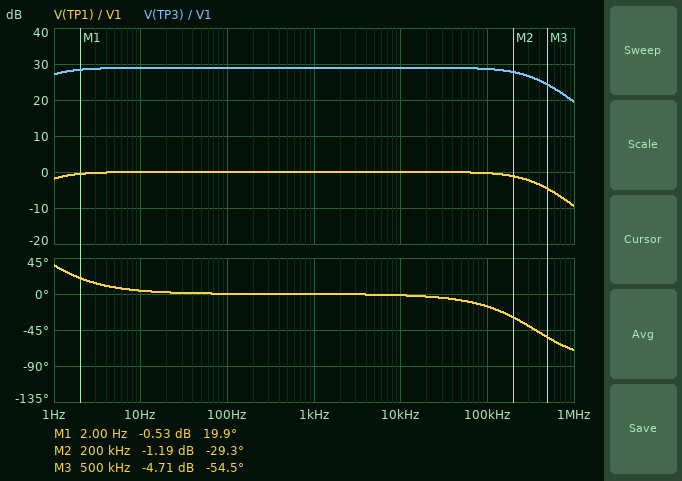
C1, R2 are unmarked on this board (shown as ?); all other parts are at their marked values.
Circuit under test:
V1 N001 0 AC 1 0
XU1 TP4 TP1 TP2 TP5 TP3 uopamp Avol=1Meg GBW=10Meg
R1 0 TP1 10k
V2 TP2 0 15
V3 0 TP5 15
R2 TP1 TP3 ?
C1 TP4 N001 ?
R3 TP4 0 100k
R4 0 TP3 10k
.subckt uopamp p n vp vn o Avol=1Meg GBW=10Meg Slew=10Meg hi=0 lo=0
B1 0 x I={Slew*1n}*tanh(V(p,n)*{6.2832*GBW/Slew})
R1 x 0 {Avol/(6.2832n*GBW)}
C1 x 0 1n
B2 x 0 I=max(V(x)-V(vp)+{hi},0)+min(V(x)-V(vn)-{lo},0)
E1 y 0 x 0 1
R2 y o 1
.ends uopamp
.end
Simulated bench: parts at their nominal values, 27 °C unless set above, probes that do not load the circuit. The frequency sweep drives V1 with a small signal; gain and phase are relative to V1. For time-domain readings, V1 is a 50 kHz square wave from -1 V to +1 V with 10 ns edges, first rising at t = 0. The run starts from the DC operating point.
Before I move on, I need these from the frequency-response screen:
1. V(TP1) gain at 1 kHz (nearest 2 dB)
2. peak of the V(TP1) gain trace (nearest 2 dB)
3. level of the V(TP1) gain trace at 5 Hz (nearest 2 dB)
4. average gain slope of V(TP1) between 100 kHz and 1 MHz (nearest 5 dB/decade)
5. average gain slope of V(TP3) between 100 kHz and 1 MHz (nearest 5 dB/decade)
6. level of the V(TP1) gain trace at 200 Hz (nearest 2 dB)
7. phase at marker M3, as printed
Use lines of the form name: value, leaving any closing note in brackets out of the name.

V(TP1) gain at 1 kHz: 0 dB
peak of the V(TP1) gain trace: 0 dB
level of the V(TP1) gain trace at 5 Hz: 0 dB
average gain slope of V(TP1) between 100 kHz and 1 MHz: -10 dB/decade
average gain slope of V(TP3) between 100 kHz and 1 MHz: -10 dB/decade
level of the V(TP1) gain trace at 200 Hz: 0 dB
phase at marker M3, as printed: -54.5 deg
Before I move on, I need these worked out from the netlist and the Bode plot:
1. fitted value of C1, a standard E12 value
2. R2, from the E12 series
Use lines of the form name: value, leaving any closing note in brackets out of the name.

fitted value of C1, a standard E12 value: 2.2 µF
R2, from the E12 series: 270 kΩ
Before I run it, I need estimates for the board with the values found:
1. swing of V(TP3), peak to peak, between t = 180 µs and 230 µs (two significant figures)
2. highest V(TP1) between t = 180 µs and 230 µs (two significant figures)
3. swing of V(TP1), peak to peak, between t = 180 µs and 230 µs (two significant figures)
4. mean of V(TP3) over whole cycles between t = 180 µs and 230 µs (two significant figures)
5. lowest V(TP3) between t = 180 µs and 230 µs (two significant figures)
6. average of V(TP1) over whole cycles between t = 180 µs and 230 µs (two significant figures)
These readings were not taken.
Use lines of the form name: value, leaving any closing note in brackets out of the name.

swing of V(TP3), peak to peak, between t = 180 µs and 230 µs: 15 V
highest V(TP1) between t = 180 µs and 230 µs: 540 mV
swing of V(TP1), peak to peak, between t = 180 µs and 230 µs: 540 mV
mean of V(TP3) over whole cycles between t = 180 µs and 230 µs: 7.6 V
lowest V(TP3) between t = 180 µs and 230 µs: -28 mV
average of V(TP1) over whole cycles between t = 180 µs and 230 µs: 270 mV
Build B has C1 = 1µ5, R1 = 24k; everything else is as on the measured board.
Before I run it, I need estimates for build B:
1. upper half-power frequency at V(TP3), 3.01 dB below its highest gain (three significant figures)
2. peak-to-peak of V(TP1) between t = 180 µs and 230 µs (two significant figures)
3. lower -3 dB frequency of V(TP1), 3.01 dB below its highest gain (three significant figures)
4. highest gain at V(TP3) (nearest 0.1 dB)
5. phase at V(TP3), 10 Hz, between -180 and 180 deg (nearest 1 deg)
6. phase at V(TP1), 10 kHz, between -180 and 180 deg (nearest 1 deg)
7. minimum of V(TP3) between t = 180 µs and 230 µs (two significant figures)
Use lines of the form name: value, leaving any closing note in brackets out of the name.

upper half-power frequency at V(TP3), 3.01 dB below its highest gain: 816 kHz
peak-to-peak of V(TP1) between t = 180 µs and 230 µs: 1.2 V
lower -3 dB frequency of V(TP1), 3.01 dB below its highest gain: 1.06 Hz
highest gain at V(TP3): 21.8 dB
phase at V(TP3), 10 Hz, between -180 and 180 deg: 6 deg
phase at V(TP1), 10 kHz, between -180 and 180 deg: -1 deg
minimum of V(TP3) between t = 180 µs and 230 µs: -18 mV
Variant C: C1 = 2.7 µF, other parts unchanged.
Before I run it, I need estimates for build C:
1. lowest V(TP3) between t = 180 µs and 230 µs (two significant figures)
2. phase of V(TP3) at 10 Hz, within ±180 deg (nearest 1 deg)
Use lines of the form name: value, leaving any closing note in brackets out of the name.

lowest V(TP3) between t = 180 µs and 230 µs: -23 mV
phase of V(TP3) at 10 Hz, within ±180 deg: 3 deg
